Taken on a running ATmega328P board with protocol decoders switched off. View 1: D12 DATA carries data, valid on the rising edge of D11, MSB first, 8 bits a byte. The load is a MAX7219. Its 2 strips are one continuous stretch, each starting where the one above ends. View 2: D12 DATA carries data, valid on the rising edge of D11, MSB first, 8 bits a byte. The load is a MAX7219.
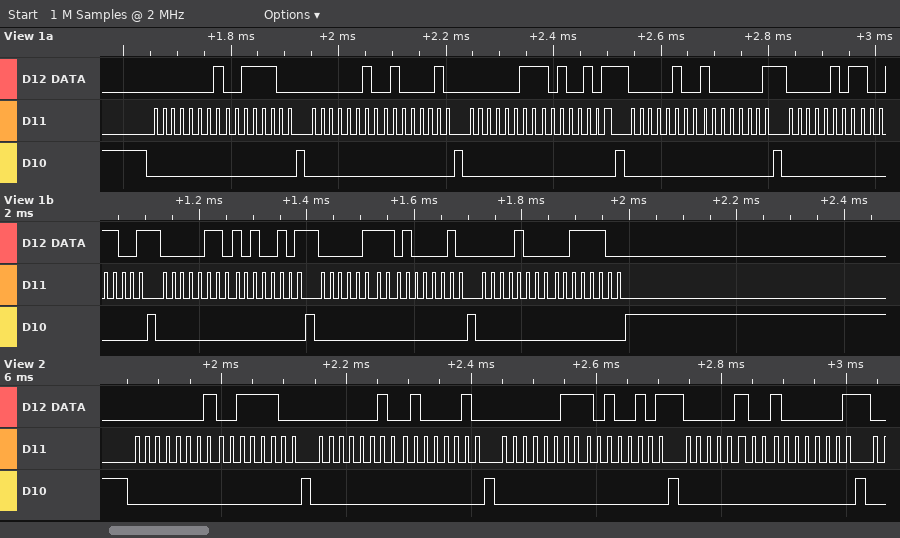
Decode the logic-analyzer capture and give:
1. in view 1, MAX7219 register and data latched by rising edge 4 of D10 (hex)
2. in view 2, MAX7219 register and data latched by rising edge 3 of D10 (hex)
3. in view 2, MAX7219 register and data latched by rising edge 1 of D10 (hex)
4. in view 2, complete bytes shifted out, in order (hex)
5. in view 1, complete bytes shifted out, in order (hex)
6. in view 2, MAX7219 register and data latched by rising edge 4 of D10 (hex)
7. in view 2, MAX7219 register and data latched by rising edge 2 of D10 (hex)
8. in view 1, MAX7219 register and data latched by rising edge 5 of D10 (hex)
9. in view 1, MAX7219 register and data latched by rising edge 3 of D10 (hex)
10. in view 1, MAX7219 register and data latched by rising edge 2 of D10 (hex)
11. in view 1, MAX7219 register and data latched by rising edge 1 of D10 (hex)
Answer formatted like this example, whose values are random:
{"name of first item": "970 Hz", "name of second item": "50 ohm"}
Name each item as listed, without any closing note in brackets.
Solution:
{"in view 1, MAX7219 register and data latched by rising edge 4 of D10": "register 0x4, data 0x81", "in view 2, MAX7219 register and data latched by rising edge 3 of D10": "register 0x3, data 0xA5", "in view 2, MAX7219 register and data latched by rising edge 1 of D10": "register 0x1, data 0x3C", "in view 2, complete bytes shifted out, in order": "01 3C 02 42 03 A5 04 81", "in view 1, complete bytes shifted out, in order": "01 3C 02 42 03 A5 04 81 05 99 06 A5 07 42 08 3C", "in view 2, MAX7219 register and data latched by rising edge 4 of D10": "register 0x4, data 0x81", "in view 2, MAX7219 register and data latched by rising edge 2 of D10": "register 0x2, data 0x42", "in view 1, MAX7219 register and data latched by rising edge 5 of D10": "register 0x5, data 0x99", "in view 1, MAX7219 register and data latched by rising edge 3 of D10": "register 0x3, data 0xA5", "in view 1, MAX7219 register and data latched by rising edge 2 of D10": "register 0x2, data 0x42", "in view 1, MAX7219 register and data latched by rising edge 1 of D10": "register 0x1, data 0x3C"}
